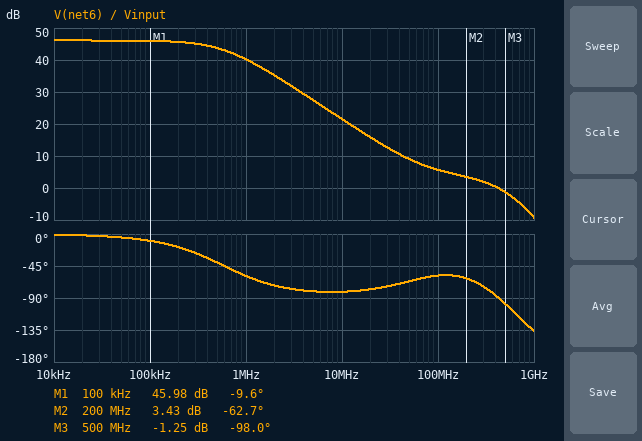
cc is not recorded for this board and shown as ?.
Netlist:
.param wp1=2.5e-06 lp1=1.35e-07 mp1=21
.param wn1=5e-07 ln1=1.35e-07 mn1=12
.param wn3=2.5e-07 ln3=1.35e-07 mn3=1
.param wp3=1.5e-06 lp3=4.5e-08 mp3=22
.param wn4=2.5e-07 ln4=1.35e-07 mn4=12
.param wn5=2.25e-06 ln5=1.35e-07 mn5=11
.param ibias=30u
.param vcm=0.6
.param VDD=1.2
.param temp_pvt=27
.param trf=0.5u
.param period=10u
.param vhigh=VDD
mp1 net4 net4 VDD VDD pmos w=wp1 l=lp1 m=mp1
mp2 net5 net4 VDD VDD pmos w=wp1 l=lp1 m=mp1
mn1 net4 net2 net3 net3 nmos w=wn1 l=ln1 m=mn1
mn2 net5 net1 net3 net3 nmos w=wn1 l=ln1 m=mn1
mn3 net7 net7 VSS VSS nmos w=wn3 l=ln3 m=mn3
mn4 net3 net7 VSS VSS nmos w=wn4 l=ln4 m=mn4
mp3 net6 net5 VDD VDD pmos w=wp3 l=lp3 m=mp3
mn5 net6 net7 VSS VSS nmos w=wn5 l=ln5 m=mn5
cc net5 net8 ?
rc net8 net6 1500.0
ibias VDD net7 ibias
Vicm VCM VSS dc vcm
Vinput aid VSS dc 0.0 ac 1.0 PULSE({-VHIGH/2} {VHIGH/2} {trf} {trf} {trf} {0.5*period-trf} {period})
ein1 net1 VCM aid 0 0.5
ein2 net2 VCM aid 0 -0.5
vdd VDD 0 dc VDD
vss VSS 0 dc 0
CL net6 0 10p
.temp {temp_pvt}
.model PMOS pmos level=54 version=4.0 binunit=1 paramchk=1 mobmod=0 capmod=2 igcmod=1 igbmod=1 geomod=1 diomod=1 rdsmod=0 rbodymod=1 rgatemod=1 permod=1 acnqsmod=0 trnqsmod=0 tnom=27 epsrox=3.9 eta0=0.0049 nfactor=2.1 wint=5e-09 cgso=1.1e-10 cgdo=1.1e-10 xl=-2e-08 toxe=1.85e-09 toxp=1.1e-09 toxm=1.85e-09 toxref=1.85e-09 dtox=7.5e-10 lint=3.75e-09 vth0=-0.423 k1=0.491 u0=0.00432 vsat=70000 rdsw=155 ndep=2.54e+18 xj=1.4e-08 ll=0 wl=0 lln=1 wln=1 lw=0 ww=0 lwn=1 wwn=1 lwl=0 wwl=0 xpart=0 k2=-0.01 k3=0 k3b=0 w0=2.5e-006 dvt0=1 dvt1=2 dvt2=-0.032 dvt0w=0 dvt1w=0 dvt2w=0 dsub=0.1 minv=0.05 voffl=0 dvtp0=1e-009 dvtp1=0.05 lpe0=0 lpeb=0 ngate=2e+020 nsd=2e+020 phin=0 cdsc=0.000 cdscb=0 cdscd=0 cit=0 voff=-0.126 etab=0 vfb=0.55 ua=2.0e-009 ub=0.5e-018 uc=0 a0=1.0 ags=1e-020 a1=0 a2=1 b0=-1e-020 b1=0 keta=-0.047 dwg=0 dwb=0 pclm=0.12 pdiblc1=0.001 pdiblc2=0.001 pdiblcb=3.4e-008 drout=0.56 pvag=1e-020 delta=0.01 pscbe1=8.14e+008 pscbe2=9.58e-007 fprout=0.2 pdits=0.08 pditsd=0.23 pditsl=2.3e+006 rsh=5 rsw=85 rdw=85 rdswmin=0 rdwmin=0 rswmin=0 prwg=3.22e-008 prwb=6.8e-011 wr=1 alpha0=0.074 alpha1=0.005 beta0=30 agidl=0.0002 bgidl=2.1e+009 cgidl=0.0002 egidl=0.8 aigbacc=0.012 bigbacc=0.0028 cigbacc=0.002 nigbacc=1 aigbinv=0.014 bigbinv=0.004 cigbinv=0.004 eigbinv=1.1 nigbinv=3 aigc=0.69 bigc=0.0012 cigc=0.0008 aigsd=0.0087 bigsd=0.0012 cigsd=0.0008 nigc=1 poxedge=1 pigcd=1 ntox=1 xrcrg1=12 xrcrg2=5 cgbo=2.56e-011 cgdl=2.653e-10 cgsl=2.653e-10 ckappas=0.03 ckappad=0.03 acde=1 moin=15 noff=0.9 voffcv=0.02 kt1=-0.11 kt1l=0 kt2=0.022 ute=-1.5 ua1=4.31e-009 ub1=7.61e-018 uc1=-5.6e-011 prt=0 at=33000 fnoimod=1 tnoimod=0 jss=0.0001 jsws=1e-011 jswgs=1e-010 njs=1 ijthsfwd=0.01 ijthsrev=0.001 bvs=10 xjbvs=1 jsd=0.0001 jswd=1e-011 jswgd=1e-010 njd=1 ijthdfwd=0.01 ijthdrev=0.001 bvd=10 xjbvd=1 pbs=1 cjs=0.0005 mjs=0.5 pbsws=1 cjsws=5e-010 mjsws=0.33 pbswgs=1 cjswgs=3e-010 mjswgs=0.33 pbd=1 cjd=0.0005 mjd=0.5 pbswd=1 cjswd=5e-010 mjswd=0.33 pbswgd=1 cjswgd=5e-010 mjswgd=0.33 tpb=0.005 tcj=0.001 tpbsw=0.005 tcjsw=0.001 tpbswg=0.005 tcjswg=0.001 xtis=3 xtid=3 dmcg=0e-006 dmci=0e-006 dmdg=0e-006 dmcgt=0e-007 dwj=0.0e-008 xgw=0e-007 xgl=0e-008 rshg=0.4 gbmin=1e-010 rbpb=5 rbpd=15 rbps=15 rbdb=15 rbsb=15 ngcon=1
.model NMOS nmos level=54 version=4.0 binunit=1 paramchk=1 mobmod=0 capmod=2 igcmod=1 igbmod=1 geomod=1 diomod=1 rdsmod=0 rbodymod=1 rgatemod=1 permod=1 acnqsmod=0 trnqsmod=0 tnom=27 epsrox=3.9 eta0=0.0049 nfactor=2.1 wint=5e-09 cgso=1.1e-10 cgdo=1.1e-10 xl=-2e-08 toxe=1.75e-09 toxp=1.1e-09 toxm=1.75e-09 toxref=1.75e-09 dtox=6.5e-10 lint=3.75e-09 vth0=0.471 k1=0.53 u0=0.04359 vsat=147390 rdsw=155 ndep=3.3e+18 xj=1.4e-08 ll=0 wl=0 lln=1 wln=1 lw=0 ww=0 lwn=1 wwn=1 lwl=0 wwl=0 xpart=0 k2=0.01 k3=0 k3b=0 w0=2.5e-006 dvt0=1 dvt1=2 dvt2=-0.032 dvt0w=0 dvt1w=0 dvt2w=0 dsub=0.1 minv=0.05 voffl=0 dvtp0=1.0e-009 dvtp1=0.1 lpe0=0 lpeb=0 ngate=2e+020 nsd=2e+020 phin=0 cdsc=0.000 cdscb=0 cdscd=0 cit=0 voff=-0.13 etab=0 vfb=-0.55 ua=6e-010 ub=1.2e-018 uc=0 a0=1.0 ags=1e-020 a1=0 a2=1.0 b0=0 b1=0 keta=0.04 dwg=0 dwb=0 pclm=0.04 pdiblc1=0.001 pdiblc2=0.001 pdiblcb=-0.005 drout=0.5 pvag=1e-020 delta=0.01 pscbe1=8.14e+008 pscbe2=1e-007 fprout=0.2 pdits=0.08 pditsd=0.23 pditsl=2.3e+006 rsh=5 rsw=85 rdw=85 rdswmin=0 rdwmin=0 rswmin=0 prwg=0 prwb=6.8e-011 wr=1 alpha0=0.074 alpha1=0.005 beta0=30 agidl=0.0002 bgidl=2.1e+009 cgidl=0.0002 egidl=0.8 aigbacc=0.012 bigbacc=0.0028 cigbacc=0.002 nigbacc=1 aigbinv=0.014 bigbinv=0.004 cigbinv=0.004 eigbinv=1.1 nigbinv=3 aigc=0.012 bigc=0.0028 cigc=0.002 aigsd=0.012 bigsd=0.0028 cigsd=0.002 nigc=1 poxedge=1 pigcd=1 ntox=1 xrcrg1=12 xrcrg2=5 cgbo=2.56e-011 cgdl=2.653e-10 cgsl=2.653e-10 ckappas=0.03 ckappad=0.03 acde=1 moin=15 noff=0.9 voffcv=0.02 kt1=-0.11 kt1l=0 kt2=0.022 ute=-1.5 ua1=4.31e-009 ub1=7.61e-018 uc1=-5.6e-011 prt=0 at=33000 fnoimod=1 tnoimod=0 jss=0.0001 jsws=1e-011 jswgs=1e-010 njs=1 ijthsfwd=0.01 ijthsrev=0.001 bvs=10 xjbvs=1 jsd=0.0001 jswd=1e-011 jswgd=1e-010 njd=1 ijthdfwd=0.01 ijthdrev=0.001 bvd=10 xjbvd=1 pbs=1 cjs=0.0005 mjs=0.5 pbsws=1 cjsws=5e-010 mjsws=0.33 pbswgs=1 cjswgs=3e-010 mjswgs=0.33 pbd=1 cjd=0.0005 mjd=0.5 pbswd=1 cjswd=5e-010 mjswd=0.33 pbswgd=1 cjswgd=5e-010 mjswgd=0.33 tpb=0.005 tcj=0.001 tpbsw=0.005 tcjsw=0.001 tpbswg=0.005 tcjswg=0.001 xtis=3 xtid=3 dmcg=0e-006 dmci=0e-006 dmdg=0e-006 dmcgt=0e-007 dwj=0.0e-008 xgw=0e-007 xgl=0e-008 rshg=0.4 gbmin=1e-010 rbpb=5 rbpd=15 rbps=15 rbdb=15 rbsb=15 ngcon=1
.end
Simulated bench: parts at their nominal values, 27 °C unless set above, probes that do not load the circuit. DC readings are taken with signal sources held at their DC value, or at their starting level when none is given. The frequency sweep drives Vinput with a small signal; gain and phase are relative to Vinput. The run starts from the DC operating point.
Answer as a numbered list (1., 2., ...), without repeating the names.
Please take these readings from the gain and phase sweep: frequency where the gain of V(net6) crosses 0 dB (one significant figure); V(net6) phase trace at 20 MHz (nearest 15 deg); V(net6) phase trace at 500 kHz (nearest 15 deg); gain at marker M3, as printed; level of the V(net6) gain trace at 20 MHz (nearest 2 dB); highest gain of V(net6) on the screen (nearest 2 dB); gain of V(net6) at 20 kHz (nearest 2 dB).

1. 400 MHz
2. -75 deg
3. -45 deg
4. -1.25 dB
5. 16 dB
6. 46 dB
7. 46 dB
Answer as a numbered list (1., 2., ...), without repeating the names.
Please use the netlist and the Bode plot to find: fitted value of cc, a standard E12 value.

1. 1.5 pF
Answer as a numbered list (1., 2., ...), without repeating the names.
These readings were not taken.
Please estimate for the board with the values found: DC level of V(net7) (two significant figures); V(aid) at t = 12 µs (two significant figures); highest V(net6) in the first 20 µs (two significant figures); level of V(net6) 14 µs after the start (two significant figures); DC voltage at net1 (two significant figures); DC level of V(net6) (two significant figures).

1. 710 mV
2. 600 mV
3. 1.1 V
4. 1.1 V
5. 600 mV
6. 320 mV
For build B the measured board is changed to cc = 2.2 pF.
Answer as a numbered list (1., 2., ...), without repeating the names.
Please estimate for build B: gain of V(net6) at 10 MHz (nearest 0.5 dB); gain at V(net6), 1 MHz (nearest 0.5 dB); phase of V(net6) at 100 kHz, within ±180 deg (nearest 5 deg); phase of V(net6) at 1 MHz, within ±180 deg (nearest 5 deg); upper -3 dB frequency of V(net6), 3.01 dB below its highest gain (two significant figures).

1. 18.5 dB
2. 37.5 dB
3. -15 deg
4. -65 deg
5. 400 kHz
